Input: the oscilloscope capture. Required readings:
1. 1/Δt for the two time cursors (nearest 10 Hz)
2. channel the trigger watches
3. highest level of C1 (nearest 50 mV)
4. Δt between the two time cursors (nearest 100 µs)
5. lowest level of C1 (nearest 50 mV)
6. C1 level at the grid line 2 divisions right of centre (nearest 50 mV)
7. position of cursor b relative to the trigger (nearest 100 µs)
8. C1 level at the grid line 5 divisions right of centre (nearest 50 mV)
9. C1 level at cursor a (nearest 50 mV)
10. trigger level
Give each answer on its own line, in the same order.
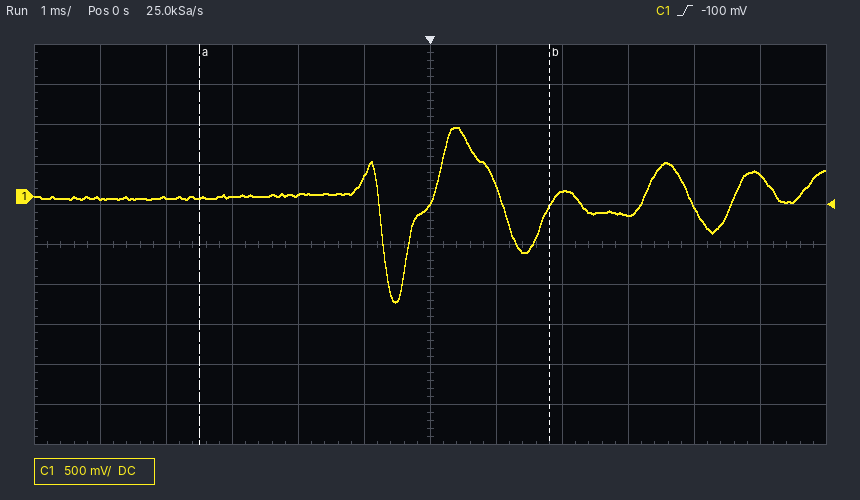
190 Hz
C1
850 mV
5.3 ms
-1.30 V
50 mV
+1.8 ms
250 mV
0 mV
-100 mV
